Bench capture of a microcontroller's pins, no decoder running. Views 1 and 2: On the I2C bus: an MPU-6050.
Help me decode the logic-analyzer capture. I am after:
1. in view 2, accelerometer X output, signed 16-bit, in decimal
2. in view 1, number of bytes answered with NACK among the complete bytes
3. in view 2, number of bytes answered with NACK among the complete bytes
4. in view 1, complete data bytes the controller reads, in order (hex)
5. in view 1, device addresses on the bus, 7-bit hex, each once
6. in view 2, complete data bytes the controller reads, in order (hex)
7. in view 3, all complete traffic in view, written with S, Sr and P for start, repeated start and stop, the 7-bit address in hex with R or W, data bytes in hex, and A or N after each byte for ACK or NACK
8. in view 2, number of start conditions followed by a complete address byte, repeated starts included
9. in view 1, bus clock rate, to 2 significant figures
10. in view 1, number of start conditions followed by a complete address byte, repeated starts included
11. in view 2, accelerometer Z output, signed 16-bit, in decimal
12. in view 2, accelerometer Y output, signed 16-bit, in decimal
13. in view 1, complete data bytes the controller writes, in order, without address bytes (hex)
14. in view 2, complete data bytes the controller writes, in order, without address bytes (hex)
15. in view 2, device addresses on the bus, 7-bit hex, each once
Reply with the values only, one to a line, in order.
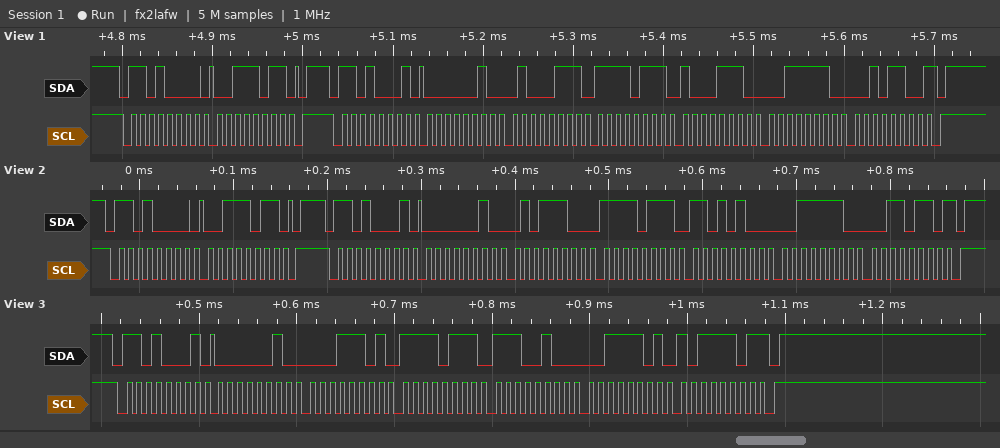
604
1
1
02 47 F7 8E 3E 2C
0x68
02 5C F7 D4 3E 36
S 68R A 02 A 1D A F7 A E4 A 3D A BD N P
2
100 kHz
2
15926
-2092
3B
3B
0x68
